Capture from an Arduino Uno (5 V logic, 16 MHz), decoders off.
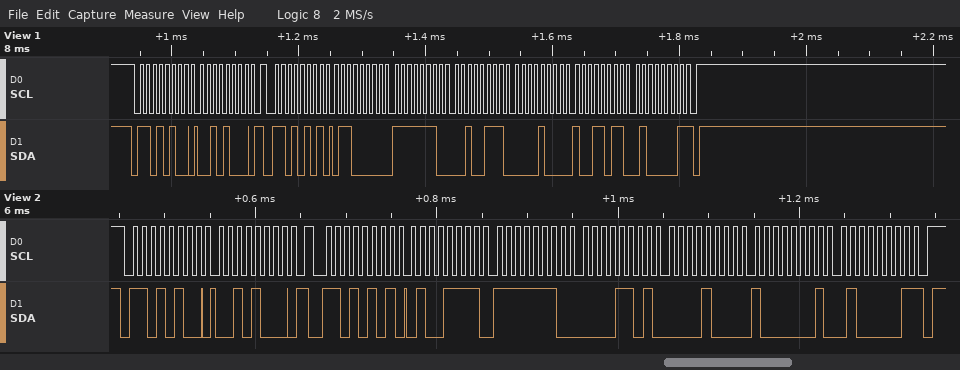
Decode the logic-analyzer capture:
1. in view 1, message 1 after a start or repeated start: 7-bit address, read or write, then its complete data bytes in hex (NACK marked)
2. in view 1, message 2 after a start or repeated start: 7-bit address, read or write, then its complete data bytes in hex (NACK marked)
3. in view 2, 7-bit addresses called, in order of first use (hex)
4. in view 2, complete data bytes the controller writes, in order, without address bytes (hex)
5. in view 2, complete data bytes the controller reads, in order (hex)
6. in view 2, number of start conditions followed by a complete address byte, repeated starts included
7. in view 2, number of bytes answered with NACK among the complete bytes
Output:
0x6A write: 28
0x6A read: 60 FE 27 08 9B 41 NACK
0x6A
28
4F FE 0D 08 81 41
2
1
